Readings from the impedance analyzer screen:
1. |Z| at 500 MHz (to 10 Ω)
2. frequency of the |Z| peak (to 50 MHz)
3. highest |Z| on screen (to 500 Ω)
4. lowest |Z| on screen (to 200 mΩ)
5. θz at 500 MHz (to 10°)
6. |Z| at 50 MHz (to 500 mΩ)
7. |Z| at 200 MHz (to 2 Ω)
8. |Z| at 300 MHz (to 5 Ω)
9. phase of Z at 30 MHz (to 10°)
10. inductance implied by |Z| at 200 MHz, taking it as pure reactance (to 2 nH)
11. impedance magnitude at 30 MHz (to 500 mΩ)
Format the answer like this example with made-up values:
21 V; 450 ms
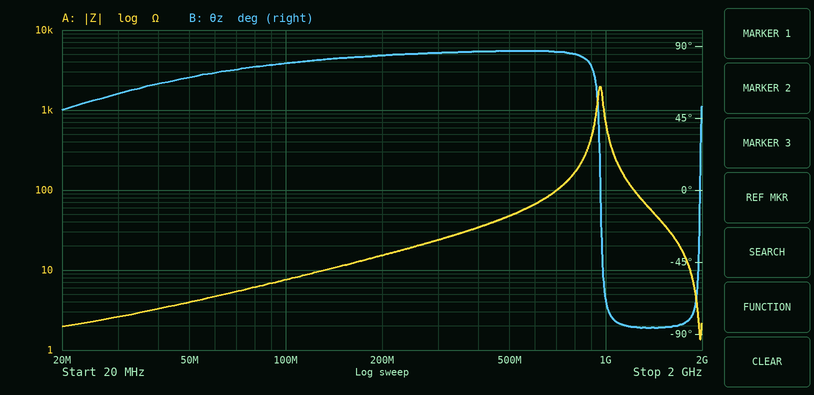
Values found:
50 Ω; 950 MHz; 2.0 kΩ; 1.4 Ω; 90°; 4.0 Ω; 16 Ω; 25 Ω; 60°; 12 nH; 2.5 Ω
